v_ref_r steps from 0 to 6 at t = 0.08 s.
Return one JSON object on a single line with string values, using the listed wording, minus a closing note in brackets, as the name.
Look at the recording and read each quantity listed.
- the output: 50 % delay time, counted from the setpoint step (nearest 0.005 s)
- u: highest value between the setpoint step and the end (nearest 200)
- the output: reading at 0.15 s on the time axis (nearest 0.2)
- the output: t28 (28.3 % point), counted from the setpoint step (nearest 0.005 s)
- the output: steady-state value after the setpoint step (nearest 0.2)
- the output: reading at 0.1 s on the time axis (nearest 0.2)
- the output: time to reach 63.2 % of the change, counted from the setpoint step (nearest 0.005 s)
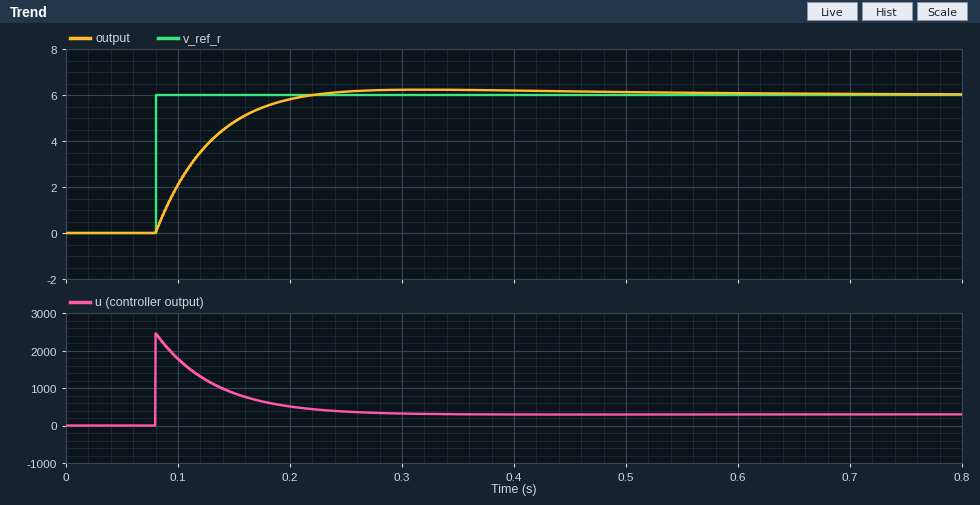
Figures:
{"the output: 50 % delay time, counted from the setpoint step": "0.030 s", "u: highest value between the setpoint step and the end": "2400", "the output: reading at 0.15 s on the time axis": "4.8", "the output: t28 (28.3 % point), counted from the setpoint step": "0.015 s", "the output: steady-state value after the setpoint step": "6.0", "the output: reading at 0.1 s on the time axis": "2.2", "the output: time to reach 63.2 % of the change, counted from the setpoint step": "0.045 s"}
